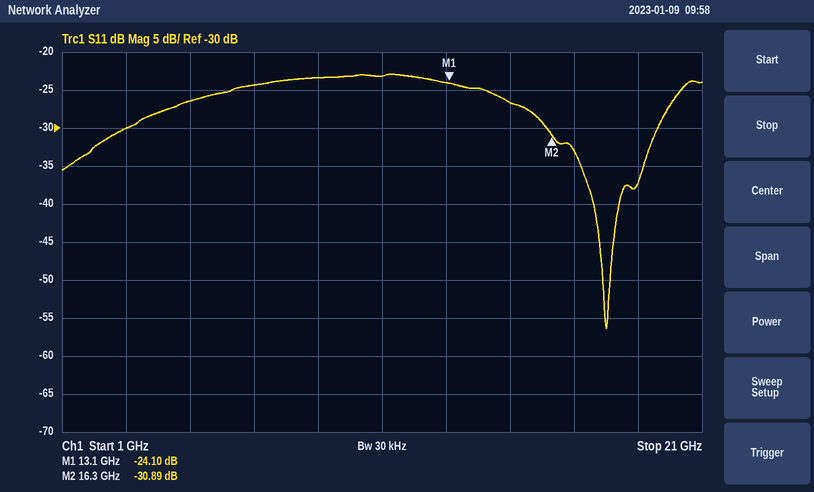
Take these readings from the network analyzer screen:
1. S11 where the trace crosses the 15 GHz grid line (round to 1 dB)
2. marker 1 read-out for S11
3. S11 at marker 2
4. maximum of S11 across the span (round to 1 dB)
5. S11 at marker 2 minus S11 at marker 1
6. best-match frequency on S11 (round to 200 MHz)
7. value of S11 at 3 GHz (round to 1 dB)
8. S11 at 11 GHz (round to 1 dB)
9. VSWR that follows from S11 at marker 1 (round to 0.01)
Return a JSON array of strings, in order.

["-27 dB", "-24.10 dB", "-30.89 dB", "-23 dB", "-6.79 dB", "18.0 GHz", "-30 dB", "-23 dB", "1.13"]
